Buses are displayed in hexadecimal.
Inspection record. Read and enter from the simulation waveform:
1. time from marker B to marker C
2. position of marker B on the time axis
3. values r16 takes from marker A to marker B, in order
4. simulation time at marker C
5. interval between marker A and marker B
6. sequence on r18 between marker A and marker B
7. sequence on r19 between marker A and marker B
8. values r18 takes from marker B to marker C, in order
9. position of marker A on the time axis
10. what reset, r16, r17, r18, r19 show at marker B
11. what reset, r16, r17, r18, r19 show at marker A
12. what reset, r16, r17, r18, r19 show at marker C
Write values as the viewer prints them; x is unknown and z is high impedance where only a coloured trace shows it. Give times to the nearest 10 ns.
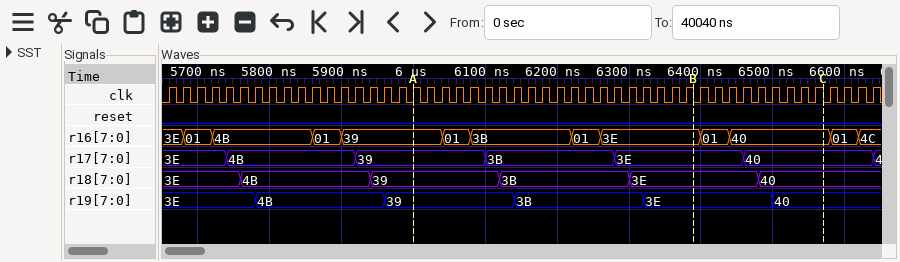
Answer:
180 ns
6390 ns
39, 01, 3B, 01, 3E
6570 ns
390 ns
39, 3B, 3E
39, 3B, 3E
3E, 40
6000 ns
reset=0, r16=3E, r17=3E, r18=3E, r19=3E
reset=0, r16=39, r17=39, r18=39, r19=39
reset=0, r16=40, r17=40, r18=40, r19=40
